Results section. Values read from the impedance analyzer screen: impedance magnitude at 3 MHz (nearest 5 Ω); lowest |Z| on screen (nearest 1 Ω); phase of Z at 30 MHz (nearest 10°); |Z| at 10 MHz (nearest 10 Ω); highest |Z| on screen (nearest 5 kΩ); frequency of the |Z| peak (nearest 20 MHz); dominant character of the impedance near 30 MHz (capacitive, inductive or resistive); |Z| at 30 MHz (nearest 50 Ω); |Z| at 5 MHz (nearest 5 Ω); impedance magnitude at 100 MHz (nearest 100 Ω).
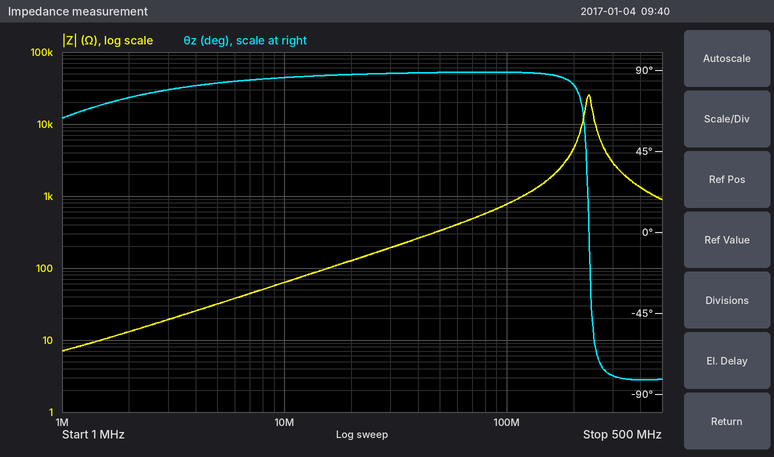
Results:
20 Ω
7 Ω
90°
60 Ω
25 kΩ
240 MHz
inductive
200 Ω
30 Ω
800 Ω
